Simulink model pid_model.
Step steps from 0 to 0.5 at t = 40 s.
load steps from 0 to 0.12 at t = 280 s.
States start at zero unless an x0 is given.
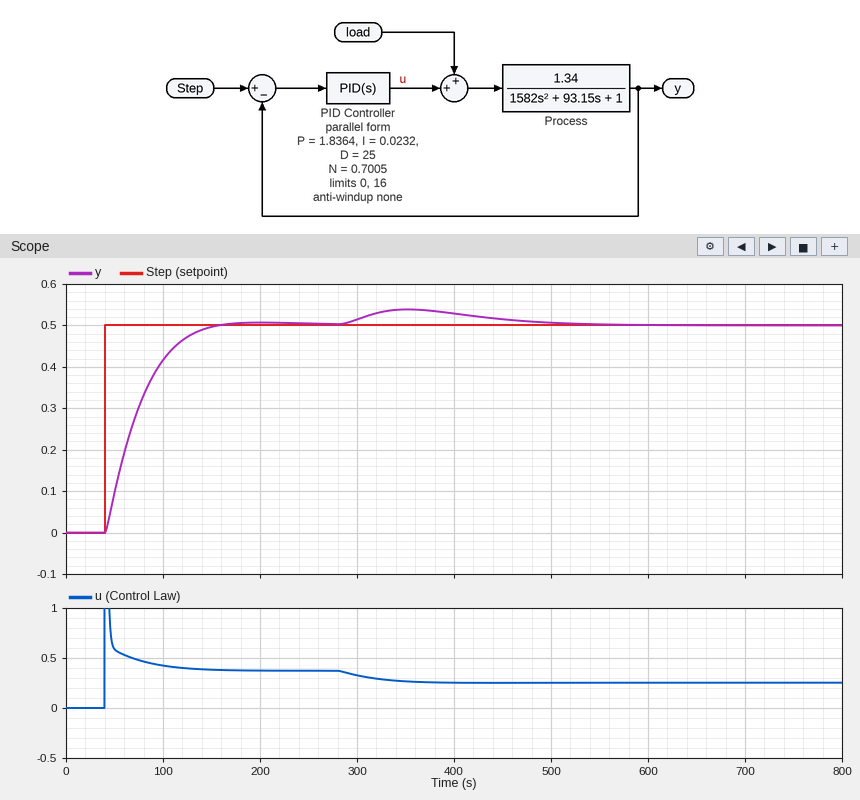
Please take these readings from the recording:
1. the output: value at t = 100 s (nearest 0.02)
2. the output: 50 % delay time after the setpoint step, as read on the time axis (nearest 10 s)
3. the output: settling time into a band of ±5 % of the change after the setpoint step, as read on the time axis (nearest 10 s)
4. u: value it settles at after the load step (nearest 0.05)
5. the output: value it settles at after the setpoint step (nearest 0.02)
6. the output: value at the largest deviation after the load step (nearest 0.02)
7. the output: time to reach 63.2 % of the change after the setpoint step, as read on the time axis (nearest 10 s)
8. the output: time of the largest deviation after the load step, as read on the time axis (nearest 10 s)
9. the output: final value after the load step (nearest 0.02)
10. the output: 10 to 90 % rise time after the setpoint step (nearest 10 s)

0.42
70 s
130 s
0.25
0.50
0.54
80 s
350 s
0.50
70 s
